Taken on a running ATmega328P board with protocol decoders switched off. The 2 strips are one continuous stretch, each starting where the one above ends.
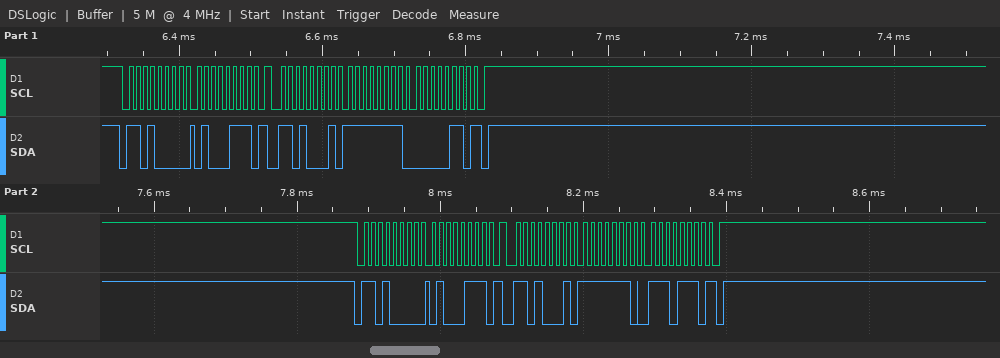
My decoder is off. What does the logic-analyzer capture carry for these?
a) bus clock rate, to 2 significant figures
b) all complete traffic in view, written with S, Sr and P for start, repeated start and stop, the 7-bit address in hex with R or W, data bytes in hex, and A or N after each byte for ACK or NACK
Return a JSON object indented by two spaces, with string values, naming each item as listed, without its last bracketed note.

{
  "bus clock rate, to 2 significant figures": "100 kHz",
  "all complete traffic in view, written with S, Sr and P for start, repeated start and stop, the 7-bit address in hex with R or W, data bytes in hex, and A or N after each byte for ACK or NACK": "S 68W A 47 A Sr 68R A FF A 06 N P S 68W A 47 A Sr 68R A FE A EE N P"
}
